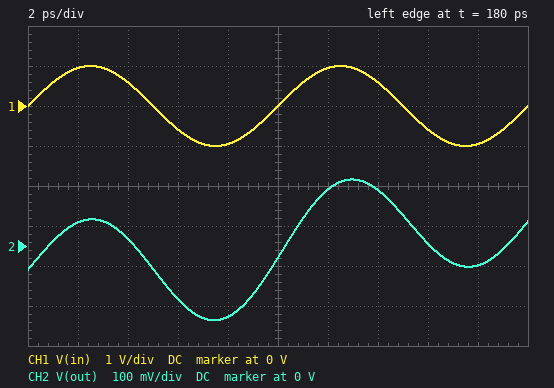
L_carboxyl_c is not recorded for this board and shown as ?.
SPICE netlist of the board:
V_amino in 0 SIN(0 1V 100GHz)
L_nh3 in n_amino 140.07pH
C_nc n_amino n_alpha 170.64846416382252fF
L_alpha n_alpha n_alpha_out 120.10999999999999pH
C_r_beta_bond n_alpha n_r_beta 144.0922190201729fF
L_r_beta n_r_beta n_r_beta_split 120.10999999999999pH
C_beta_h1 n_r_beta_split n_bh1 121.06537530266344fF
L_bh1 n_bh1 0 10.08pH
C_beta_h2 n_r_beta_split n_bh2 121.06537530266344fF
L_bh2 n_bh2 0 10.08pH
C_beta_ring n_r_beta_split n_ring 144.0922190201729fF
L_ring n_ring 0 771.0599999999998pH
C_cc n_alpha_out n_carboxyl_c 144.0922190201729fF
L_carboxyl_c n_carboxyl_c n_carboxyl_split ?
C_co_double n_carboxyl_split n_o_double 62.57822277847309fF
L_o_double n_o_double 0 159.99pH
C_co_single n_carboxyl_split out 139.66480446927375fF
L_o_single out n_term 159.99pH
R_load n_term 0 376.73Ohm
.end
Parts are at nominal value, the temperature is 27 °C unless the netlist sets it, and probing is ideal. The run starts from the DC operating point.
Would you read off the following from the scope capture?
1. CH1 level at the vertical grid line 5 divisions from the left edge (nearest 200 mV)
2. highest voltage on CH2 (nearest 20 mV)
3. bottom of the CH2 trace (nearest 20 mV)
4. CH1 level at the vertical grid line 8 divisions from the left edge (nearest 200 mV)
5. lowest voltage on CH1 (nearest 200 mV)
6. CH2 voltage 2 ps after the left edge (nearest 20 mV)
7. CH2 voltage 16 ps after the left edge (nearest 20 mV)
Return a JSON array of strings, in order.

["0 V", "160 mV", "-180 mV", "-600 mV", "-1.0 V", "60 mV", "0 V"]
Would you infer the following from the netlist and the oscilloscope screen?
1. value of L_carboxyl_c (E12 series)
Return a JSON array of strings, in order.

["100 pH"]
